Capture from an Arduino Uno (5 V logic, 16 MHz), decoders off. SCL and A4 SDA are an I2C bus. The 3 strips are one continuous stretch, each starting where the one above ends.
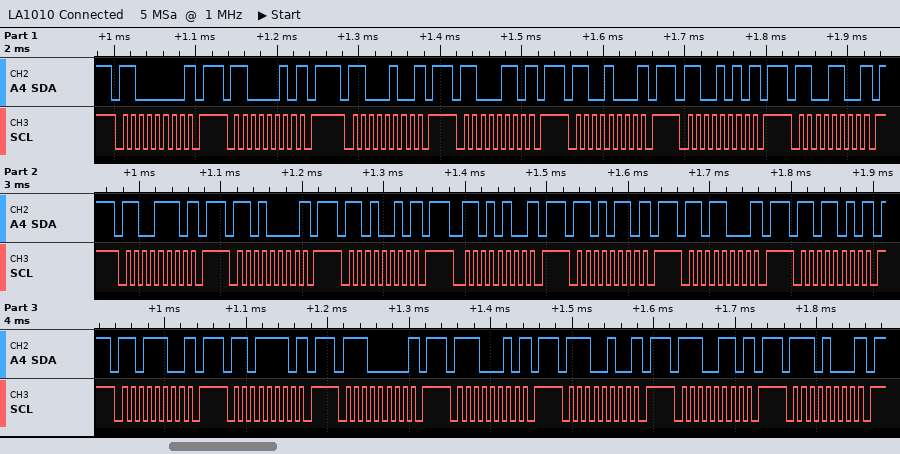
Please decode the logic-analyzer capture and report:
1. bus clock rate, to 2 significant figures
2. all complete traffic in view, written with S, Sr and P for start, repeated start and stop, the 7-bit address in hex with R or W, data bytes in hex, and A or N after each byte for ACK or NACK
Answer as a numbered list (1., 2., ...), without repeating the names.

1. 100 kHz
2. S 60W N P S 61W N P S 62W N P S 63W N P S 64W N P S 65W N P S 66W N P S 67W N P S 68W N P S 69W N P S 6AW N P S 6BW N P S 6CW N P S 6DW N P S 6EW N P S 6FW N P S 70W N P S 71W N P S 72W N P S 73W N P S 74W N P
